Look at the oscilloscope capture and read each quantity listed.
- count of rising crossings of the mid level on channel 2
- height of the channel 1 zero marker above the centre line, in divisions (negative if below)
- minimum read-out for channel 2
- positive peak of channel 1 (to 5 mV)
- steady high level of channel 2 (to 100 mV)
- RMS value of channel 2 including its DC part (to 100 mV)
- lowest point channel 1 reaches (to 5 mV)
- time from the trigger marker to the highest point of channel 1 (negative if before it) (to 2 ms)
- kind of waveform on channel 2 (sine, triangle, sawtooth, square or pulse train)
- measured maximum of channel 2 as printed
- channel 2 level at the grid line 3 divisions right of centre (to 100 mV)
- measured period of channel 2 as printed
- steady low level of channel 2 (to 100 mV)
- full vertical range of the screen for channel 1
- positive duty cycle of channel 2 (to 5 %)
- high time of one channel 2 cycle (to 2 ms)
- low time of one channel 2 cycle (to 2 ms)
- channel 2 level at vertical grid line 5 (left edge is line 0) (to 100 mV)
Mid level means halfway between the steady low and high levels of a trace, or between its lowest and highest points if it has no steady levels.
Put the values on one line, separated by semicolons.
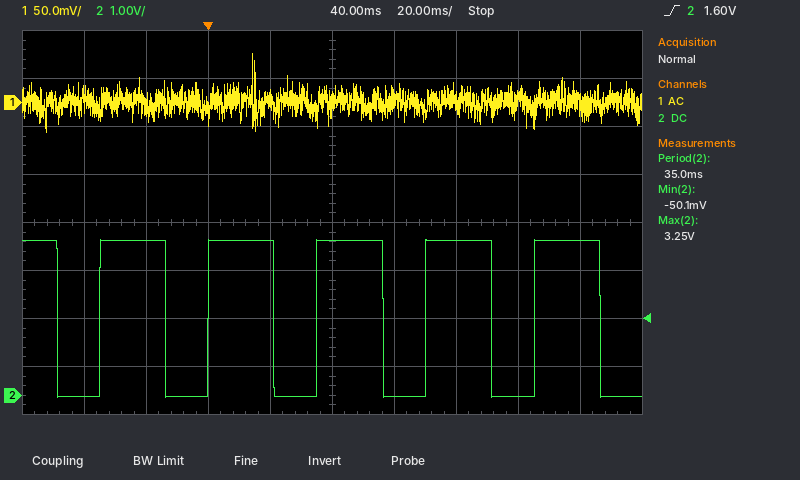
5; +2.5 div; -50.1 mV; 50 mV; 3.2 V; 2.5 V; -30 mV; +14 ms; pulse train; 3.25 V; 0.0 V; 35.0 ms; 0.0 V; 400 mV; 60 %; 22 ms; 14 ms; 3.2 V
